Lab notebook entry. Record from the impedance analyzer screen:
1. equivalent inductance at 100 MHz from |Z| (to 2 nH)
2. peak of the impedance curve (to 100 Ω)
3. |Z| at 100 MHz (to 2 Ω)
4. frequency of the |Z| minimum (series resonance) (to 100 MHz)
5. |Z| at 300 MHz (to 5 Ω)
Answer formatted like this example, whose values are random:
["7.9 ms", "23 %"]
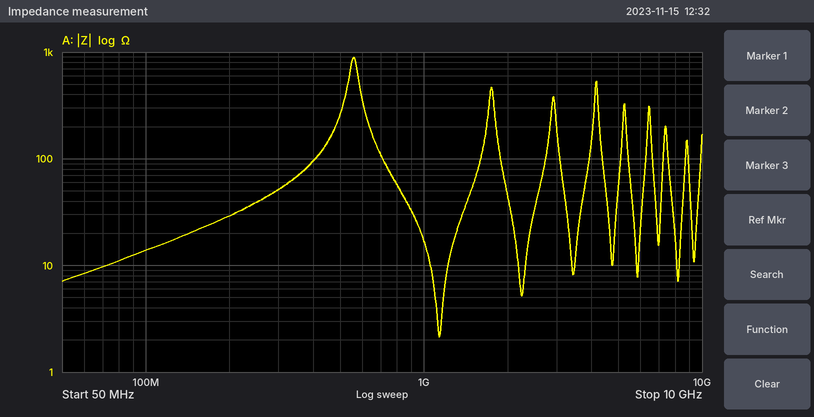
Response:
["22 nH", "900 Ω", "14 Ω", "1.1 GHz", "50 Ω"]
